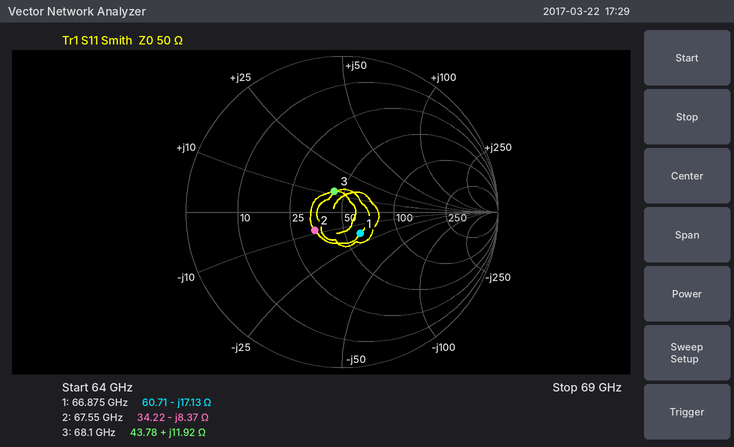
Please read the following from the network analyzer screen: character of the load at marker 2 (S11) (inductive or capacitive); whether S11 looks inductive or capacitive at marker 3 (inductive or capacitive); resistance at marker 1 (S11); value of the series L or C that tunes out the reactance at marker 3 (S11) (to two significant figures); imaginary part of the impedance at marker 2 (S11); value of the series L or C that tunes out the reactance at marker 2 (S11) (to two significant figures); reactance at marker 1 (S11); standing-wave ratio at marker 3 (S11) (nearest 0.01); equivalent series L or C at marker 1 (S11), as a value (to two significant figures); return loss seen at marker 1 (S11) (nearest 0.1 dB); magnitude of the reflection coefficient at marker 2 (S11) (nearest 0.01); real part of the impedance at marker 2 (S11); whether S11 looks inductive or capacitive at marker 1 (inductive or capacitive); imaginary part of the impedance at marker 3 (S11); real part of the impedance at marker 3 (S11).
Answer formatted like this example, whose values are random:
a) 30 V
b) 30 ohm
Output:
a) capacitive
b) inductive
c) 60.71 Ω
d) 200 fF
e) -8.37 Ω
f) 20 pH
g) -17.13 Ω
h) 1.33
i) 140 fF
j) 14.9 dB
k) 0.21
l) 34.22 Ω
m) capacitive
n) +11.92 Ω
o) 43.78 Ω
